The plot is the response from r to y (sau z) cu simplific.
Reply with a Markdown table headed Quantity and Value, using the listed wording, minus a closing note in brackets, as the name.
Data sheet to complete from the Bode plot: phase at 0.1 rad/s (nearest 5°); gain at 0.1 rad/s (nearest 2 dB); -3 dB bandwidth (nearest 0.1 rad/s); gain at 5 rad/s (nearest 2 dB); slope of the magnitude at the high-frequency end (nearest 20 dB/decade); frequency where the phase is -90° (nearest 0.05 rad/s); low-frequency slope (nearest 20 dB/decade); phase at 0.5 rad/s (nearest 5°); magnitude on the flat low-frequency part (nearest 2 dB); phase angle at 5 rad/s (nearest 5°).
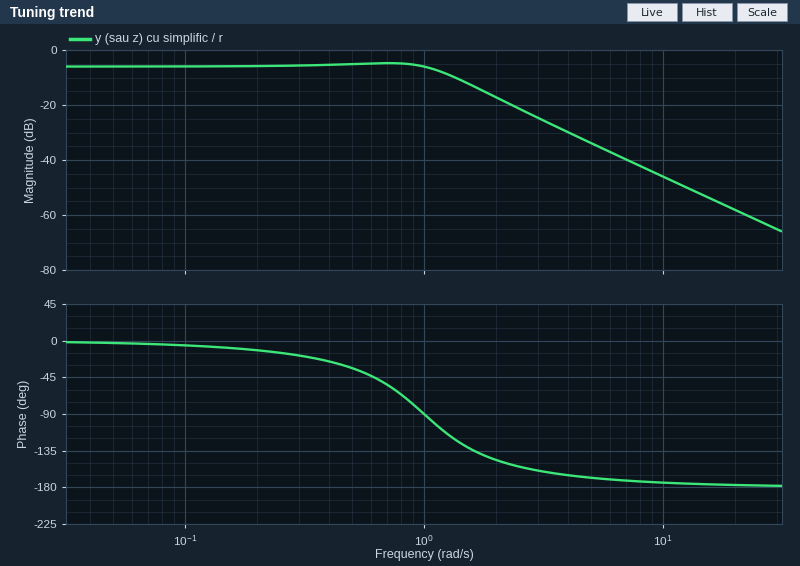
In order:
| Quantity | Value |
|---|---|
| phase at 0.1 rad/s | -5° |
| gain at 0.1 rad/s | -6 dB |
| -3 dB bandwidth | 1.3 rad/s |
| gain at 5 rad/s | -34 dB |
| slope of the magnitude at the high-frequency end | -40 dB/decade |
| frequency where the phase is -90° | 1.00 rad/s |
| low-frequency slope | 0 dB/decade |
| phase at 0.5 rad/s | -35° |
| magnitude on the flat low-frequency part | -6 dB |
| phase angle at 5 rad/s | -170° |
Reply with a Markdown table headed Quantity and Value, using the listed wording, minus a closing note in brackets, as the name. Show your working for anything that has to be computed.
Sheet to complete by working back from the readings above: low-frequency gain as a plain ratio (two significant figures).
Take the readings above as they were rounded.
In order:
| Quantity | Value |
|---|---|
| low-frequency gain as a plain ratio | 10^(-6 / 20) = 0.50 |
